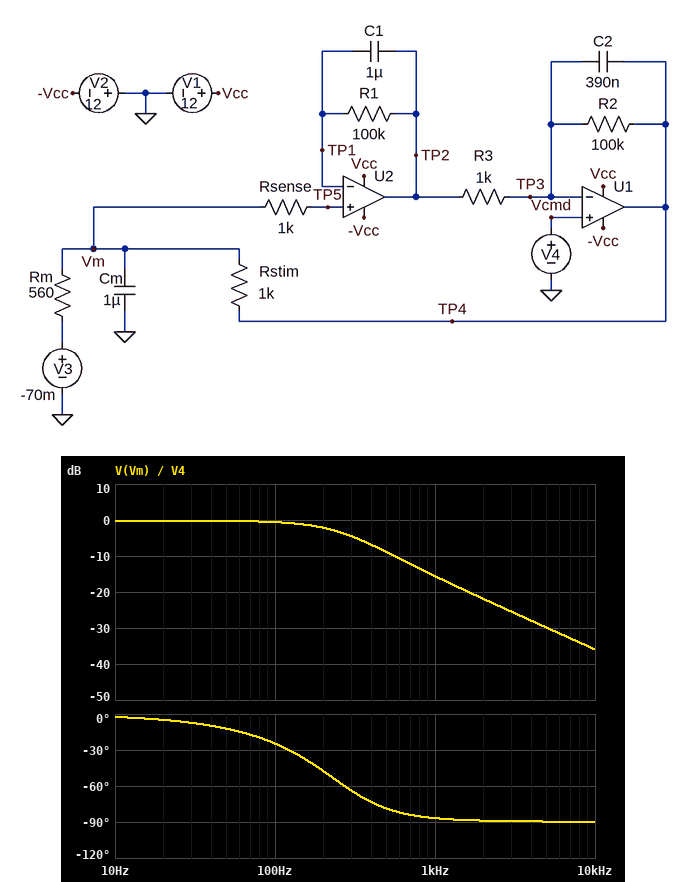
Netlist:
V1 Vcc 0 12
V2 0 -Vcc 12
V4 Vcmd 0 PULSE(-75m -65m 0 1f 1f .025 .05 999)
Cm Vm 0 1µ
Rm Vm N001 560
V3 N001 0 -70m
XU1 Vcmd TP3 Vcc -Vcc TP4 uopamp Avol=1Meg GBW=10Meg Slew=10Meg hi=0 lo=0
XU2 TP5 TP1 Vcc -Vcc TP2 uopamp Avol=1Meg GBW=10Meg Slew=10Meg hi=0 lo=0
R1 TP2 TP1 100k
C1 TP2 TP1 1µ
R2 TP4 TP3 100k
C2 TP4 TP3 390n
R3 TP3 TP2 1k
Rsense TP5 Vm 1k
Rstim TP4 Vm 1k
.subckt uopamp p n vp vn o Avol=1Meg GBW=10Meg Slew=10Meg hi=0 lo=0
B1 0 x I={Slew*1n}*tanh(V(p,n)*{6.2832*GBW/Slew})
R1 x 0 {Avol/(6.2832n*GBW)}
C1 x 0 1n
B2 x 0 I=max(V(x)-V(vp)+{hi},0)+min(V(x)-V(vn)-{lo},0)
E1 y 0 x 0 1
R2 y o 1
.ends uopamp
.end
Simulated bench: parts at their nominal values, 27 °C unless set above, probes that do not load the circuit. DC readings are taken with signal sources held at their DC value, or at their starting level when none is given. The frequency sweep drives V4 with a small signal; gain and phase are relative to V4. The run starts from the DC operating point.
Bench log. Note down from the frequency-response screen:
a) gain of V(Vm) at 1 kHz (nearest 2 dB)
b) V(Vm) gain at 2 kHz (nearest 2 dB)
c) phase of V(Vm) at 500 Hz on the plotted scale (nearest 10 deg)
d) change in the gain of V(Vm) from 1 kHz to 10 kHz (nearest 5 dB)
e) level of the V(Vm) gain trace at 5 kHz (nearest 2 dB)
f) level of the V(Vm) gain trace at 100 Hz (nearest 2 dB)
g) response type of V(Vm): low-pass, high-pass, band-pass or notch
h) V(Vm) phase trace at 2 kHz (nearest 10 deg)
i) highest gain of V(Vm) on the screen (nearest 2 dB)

-16 dB
-22 dB
-80 deg
-20 dB
-30 dB
0 dB
low-pass
-90 deg
0 dB
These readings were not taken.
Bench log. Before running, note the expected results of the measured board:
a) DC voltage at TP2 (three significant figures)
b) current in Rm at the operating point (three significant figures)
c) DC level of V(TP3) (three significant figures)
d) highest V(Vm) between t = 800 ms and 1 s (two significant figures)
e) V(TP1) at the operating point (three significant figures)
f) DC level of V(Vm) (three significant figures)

-74.9 mV
8.77 µA
-75.0 mV
-65 mV
-74.9 mV
-74.9 mV
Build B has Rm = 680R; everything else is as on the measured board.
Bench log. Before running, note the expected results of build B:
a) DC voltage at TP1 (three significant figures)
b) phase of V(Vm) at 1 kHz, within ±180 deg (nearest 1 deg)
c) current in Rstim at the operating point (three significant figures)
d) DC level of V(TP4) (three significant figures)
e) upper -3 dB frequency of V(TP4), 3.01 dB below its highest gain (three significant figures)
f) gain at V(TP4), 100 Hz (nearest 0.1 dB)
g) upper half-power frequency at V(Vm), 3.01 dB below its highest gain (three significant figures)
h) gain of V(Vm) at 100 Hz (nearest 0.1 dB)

-74.9 mV
-89 deg
7.25 µA
-82.2 mV
393 Hz
7.9 dB
286 Hz
-0.2 dB
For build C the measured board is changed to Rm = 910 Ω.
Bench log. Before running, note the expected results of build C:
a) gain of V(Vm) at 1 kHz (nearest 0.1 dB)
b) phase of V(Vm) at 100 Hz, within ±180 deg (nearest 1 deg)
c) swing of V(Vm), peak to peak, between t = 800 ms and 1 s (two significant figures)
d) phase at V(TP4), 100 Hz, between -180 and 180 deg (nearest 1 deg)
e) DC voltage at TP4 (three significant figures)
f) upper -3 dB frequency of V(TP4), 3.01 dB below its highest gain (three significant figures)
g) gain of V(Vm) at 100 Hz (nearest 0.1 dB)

-15.2 dB
-17 deg
12 mV
-1 deg
-80.4 mV
427 Hz
0.2 dB
